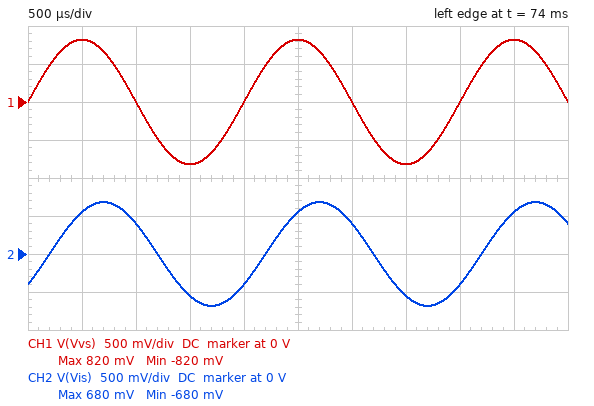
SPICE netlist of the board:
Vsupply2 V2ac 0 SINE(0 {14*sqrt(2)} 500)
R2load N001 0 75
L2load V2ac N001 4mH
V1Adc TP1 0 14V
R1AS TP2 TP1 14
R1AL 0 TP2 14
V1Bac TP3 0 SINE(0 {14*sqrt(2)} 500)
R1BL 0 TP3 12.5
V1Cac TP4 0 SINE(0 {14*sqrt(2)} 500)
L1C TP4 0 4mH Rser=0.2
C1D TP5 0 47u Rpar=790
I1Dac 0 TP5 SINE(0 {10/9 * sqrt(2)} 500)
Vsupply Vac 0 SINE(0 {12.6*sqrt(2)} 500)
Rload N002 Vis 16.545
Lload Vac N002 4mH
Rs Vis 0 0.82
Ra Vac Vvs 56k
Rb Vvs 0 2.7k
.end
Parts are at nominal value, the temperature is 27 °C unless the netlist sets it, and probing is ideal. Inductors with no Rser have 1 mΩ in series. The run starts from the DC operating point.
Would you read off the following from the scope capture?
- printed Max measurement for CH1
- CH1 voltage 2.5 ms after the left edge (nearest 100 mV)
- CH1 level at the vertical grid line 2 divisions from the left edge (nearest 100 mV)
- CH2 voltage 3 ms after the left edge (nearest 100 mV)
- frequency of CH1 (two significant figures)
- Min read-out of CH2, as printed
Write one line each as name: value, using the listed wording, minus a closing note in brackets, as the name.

printed Max measurement for CH1: 820 mV
CH1 voltage 2.5 ms after the left edge: 800 mV
CH1 level at the vertical grid line 2 divisions from the left edge: 0 V
CH2 voltage 3 ms after the left edge: 400 mV
frequency of CH1: 500 Hz
Min read-out of CH2, as printed: -680 mV
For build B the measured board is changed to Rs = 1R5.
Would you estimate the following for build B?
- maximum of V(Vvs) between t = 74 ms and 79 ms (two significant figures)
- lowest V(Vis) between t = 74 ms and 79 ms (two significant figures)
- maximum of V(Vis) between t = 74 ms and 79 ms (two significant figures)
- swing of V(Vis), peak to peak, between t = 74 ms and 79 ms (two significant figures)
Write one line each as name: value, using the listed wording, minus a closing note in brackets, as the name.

maximum of V(Vvs) between t = 74 ms and 79 ms: 820 mV
lowest V(Vis) between t = 74 ms and 79 ms: -1.2 V
maximum of V(Vis) between t = 74 ms and 79 ms: 1.2 V
swing of V(Vis), peak to peak, between t = 74 ms and 79 ms: 2.4 V
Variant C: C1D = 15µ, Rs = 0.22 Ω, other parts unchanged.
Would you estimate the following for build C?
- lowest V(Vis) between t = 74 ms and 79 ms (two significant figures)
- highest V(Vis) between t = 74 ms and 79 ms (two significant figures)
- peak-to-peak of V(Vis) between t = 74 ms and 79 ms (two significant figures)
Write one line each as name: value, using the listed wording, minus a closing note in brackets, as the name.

lowest V(Vis) between t = 74 ms and 79 ms: -190 mV
highest V(Vis) between t = 74 ms and 79 ms: 190 mV
peak-to-peak of V(Vis) between t = 74 ms and 79 ms: 370 mV
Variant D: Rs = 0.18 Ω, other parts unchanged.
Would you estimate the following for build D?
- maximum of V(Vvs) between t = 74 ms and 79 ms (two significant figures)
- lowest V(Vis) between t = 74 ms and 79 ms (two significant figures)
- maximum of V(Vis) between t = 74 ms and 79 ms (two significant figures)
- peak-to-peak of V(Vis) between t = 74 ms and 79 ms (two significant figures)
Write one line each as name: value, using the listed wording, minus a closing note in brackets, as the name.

maximum of V(Vvs) between t = 74 ms and 79 ms: 820 mV
lowest V(Vis) between t = 74 ms and 79 ms: -150 mV
maximum of V(Vis) between t = 74 ms and 79 ms: 150 mV
peak-to-peak of V(Vis) between t = 74 ms and 79 ms: 310 mV
